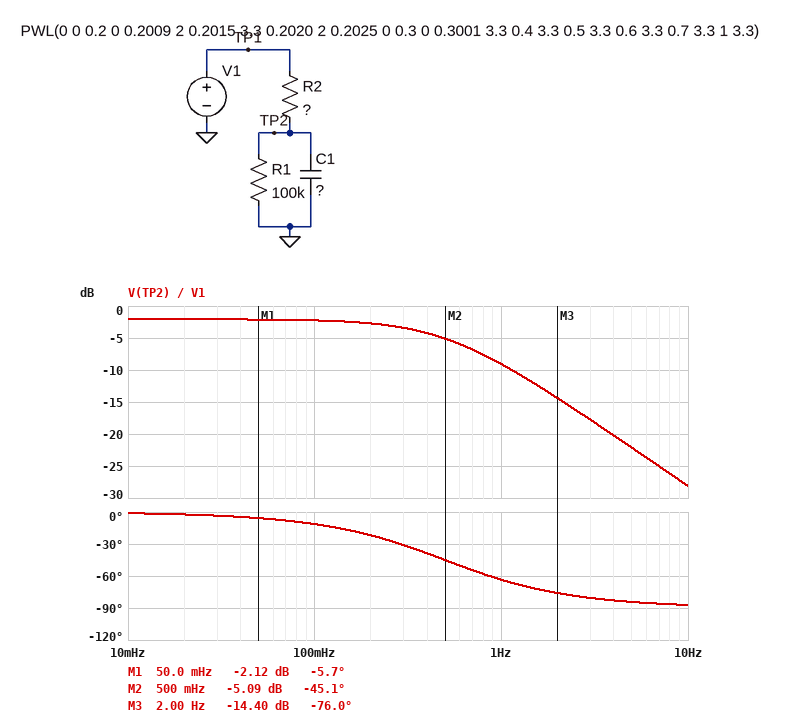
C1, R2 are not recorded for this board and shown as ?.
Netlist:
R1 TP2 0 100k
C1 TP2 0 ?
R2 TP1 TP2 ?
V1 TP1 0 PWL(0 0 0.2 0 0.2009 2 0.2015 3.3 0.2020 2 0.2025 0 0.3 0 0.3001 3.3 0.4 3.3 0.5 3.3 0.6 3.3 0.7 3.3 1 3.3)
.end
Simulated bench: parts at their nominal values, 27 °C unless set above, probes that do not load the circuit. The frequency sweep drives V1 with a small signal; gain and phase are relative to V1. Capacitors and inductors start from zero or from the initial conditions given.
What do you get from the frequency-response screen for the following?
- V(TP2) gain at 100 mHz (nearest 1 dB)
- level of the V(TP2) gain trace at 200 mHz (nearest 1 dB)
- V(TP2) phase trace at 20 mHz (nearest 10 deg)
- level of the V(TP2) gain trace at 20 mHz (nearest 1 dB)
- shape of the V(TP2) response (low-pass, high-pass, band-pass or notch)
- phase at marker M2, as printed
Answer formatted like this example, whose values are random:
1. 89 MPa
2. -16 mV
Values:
1. -2 dB
2. -3 dB
3. 0 deg
4. -2 dB
5. low-pass
6. -45.1 deg
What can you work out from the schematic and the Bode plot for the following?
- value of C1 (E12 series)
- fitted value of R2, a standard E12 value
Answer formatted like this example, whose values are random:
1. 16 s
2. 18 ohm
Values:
1. 15 µF
2. 27 kΩ
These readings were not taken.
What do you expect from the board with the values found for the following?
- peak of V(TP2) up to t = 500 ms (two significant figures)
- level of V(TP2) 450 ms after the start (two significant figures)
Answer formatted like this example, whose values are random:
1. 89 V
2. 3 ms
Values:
1. 1.2 V
2. 980 mV
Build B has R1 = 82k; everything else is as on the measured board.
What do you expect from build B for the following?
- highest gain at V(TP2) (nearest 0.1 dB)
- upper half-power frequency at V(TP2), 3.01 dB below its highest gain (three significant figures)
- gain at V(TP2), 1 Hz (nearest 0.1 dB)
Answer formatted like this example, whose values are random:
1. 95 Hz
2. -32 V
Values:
1. -2.5 dB
2. 522 mHz
3. -9.2 dB
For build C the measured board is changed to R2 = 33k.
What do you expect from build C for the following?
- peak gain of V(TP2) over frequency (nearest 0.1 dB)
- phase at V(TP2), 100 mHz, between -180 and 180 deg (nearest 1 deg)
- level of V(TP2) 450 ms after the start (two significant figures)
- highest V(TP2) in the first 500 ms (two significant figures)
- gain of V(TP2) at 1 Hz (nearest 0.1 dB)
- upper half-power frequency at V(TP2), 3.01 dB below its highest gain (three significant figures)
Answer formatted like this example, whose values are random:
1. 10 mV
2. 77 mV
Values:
1. -2.5 dB
2. -13 deg
3. 830 mV
4. 1.0 V
5. -10.6 dB
6. 428 mHz
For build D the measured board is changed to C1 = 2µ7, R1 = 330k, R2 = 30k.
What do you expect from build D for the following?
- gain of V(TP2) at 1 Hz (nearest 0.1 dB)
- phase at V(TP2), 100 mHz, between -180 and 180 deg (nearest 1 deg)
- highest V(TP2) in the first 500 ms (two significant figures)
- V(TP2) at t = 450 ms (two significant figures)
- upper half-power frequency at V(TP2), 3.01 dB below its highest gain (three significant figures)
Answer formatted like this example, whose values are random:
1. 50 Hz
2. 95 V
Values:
1. -1.6 dB
2. -3 deg
3. 2.8 V
4. 2.6 V
5. 2.14 Hz
